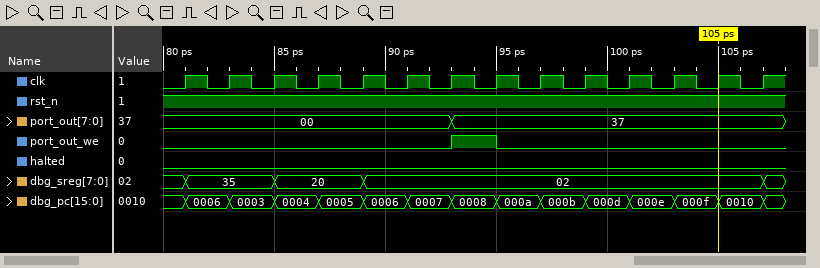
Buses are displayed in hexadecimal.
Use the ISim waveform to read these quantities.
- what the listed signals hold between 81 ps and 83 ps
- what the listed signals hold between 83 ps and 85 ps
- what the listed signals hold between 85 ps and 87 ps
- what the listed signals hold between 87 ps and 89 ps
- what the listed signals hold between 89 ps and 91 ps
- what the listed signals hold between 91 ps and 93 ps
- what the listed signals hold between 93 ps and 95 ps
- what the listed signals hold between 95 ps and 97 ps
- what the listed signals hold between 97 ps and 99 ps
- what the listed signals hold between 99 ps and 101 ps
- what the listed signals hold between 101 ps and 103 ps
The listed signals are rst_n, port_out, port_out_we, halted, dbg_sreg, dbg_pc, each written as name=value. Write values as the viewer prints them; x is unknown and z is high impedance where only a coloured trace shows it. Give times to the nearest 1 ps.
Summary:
rst_n=1, port_out=00, port_out_we=0, halted=0, dbg_sreg=35, dbg_pc=0006
rst_n=1, port_out=00, port_out_we=0, halted=0, dbg_sreg=35, dbg_pc=0003
rst_n=1, port_out=00, port_out_we=0, halted=0, dbg_sreg=20, dbg_pc=0004
rst_n=1, port_out=00, port_out_we=0, halted=0, dbg_sreg=20, dbg_pc=0005
rst_n=1, port_out=00, port_out_we=0, halted=0, dbg_sreg=02, dbg_pc=0006
rst_n=1, port_out=00, port_out_we=0, halted=0, dbg_sreg=02, dbg_pc=0007
rst_n=1, port_out=37, port_out_we=1, halted=0, dbg_sreg=02, dbg_pc=0008
rst_n=1, port_out=37, port_out_we=0, halted=0, dbg_sreg=02, dbg_pc=000a
rst_n=1, port_out=37, port_out_we=0, halted=0, dbg_sreg=02, dbg_pc=000b
rst_n=1, port_out=37, port_out_we=0, halted=0, dbg_sreg=02, dbg_pc=000d
rst_n=1, port_out=37, port_out_we=0, halted=0, dbg_sreg=02, dbg_pc=000e
